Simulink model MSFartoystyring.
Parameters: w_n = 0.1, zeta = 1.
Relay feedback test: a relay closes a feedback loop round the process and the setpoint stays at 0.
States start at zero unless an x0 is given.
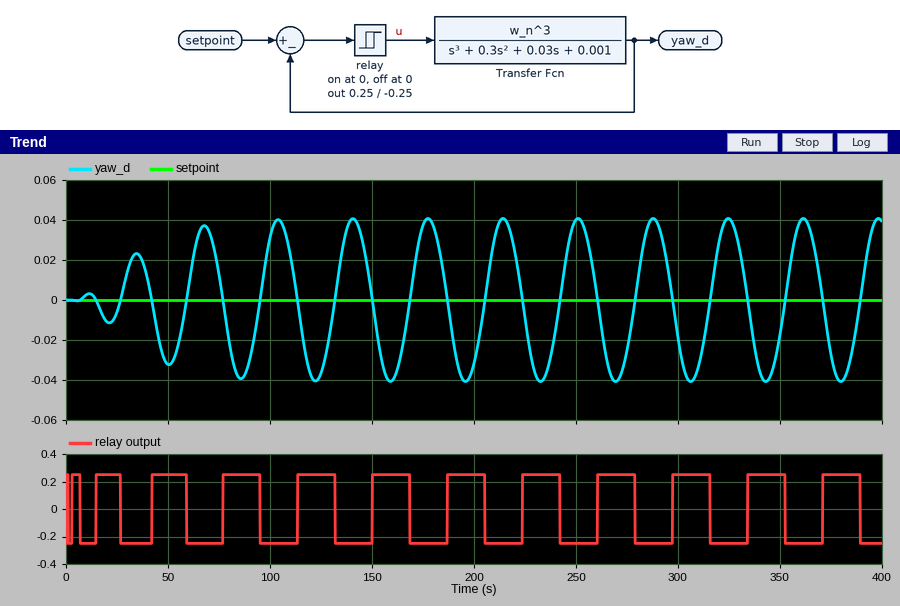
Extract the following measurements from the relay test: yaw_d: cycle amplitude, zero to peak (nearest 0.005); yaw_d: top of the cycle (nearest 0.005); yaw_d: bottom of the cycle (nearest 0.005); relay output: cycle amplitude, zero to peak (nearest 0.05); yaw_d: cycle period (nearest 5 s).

0.040
0.040
-0.040
0.25
35 s
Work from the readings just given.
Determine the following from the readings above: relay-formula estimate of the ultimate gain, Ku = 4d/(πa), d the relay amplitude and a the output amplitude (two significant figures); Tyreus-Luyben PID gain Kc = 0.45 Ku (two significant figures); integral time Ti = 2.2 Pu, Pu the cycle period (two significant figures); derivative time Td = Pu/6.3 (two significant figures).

8.0
3.6
77 s
5.6 s
